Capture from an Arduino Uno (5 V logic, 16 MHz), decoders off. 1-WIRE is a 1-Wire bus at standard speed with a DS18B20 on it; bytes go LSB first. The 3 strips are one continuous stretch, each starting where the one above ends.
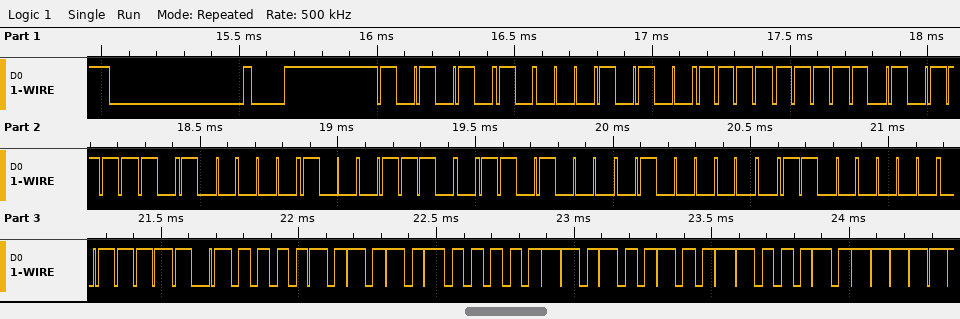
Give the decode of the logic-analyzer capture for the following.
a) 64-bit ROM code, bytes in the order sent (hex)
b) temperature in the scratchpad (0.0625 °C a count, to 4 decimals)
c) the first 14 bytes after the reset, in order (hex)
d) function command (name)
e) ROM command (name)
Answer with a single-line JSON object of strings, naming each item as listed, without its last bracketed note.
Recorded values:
{"64-bit ROM code, bytes in the order sent": "28 FF F5 05 71 16 02 03", "temperature in the scratchpad": "85.0000 °C", "the first 14 bytes after the reset, in order": "55 28 FF F5 05 71 16 02 03 BE 50 05 4B 46", "function command": "Read Scratchpad", "ROM command": "Match ROM"}
